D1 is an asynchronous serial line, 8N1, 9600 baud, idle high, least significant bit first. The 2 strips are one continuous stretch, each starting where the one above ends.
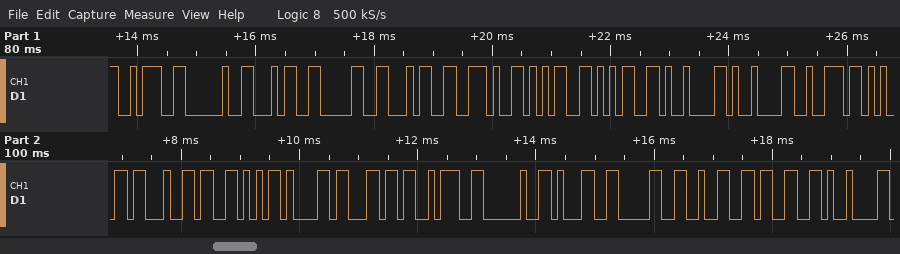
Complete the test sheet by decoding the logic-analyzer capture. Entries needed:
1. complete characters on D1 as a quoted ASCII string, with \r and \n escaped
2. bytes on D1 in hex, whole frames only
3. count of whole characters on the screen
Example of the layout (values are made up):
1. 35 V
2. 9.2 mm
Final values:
1. ": 404.55\t\tredVal: 1023\t"
2. 3A 20 34 30 34 2E 35 35 09 09 72 65 64 56 61 6C 3A 20 31 30 32 33 09
3. 23
